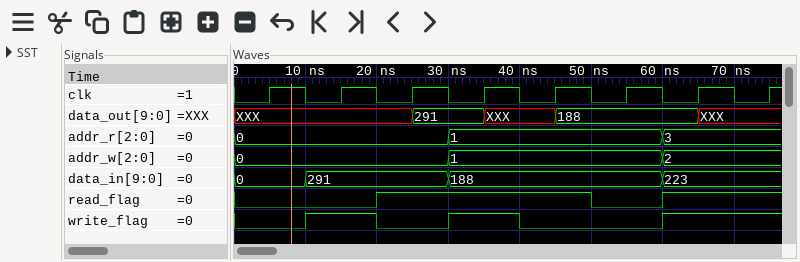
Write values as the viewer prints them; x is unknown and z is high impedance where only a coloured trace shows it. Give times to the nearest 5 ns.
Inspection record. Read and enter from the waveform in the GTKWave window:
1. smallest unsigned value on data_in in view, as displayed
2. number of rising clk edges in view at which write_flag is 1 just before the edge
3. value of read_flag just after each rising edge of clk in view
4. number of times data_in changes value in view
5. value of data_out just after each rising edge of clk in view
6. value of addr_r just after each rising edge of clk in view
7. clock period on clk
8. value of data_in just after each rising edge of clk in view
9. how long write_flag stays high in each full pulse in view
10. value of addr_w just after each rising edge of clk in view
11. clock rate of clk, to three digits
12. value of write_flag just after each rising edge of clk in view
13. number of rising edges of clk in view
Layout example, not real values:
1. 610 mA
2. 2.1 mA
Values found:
1. 0
2. 4
3. 0 0 1 1 1 0 1 1
4. 3
5. XXX, XXX, 291, XXX, 188, 188, XXX, XXX
6. 0, 0, 0, 1, 1, 1, 3, 3
7. 10 ns
8. 0, 291, 291, 188, 188, 188, 223, 223
9. 10 ns, 10 ns
10. 0, 0, 0, 1, 1, 1, 2, 2
11. 100 MHz
12. 0 1 0 1 0 0 1 1
13. 8
